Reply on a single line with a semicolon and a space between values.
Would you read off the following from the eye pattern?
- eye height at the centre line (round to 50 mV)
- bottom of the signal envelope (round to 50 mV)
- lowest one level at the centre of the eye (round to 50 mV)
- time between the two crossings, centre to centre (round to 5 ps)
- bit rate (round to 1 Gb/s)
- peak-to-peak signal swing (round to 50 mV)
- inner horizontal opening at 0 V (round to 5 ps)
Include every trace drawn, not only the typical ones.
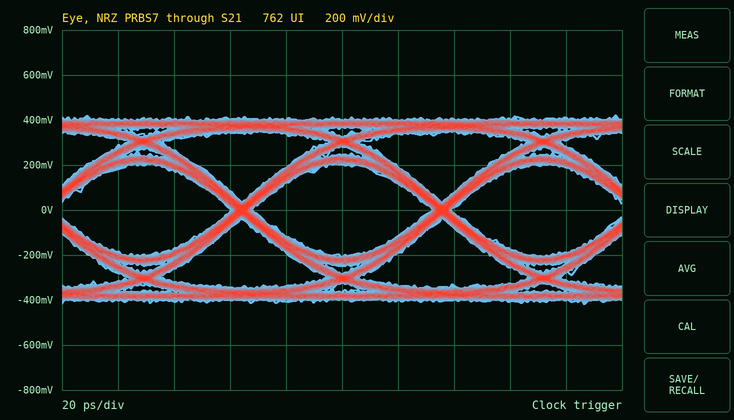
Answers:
400 mV; -400 mV; 200 mV; 70 ps; 14 Gb/s; 850 mV; 65 ps
